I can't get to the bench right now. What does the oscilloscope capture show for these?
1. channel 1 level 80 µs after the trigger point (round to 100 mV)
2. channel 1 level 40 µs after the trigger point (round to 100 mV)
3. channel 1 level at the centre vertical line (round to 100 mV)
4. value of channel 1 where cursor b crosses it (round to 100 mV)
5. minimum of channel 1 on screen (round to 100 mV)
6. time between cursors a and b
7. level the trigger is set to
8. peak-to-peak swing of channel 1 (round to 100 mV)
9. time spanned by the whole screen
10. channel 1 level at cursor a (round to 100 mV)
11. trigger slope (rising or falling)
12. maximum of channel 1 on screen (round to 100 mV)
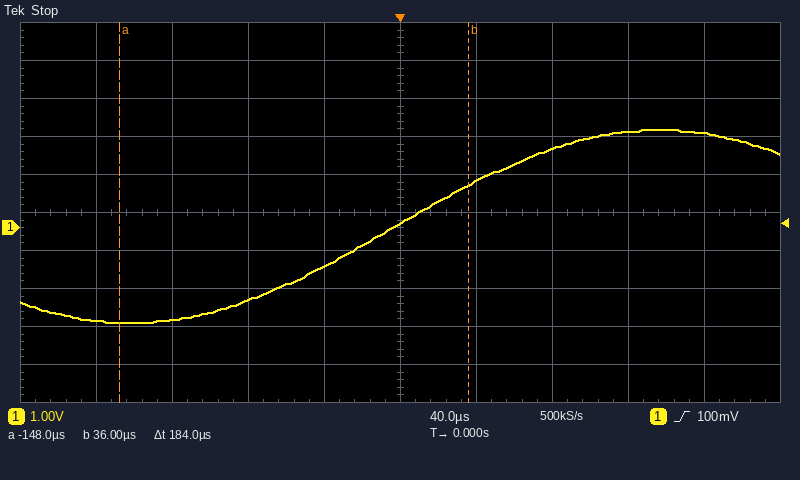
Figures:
2.1 V
1.2 V
100 mV
1.1 V
-2.5 V
184 µs
100 mV
5.1 V
400 µs
-2.5 V
rising
2.6 V
